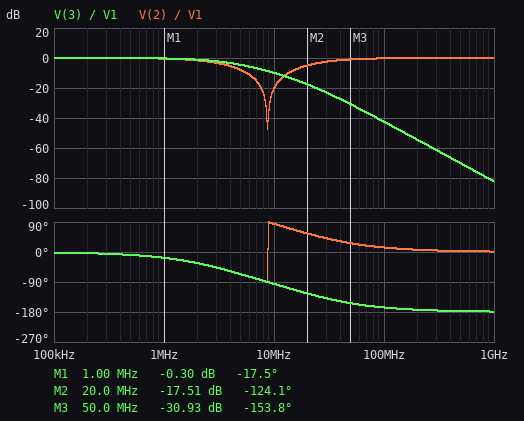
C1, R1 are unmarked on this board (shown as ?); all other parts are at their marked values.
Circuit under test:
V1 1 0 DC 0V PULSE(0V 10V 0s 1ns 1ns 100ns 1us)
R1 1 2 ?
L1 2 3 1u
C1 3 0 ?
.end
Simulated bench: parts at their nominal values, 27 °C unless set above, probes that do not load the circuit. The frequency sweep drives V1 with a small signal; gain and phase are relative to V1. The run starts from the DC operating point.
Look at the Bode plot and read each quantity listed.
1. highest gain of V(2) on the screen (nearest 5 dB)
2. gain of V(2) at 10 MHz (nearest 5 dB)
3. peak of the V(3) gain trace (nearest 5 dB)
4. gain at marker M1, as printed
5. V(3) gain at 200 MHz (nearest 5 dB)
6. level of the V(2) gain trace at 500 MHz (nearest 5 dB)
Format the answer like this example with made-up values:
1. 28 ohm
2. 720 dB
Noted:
1. 0 dB
2. -20 dB
3. 0 dB
4. -0.30 dB
5. -55 dB
6. 0 dB
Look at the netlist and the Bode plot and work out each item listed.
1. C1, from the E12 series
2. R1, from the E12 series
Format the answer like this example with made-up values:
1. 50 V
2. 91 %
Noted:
1. 330 pF
2. 150 Ω
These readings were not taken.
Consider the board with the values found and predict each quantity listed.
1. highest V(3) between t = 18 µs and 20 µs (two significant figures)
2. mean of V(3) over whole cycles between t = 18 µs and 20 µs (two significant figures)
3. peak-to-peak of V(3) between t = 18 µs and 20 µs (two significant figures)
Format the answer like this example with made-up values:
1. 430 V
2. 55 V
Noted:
1. 8.9 V
2. 1.0 V
3. 8.9 V
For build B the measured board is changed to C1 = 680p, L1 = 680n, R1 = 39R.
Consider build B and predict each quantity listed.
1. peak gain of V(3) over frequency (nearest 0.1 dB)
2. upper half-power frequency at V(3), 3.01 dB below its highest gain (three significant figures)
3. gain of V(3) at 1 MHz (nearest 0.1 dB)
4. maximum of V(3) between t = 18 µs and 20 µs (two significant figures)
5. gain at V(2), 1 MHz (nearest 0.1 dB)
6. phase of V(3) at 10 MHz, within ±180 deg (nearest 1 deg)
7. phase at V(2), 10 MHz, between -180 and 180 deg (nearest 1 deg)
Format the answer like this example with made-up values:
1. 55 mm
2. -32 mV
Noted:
1. 0.3 dB
2. 8.14 MHz
3. 0 dB
4. 11 V
5. -0.1 dB
6. -116 deg
7. 64 deg
